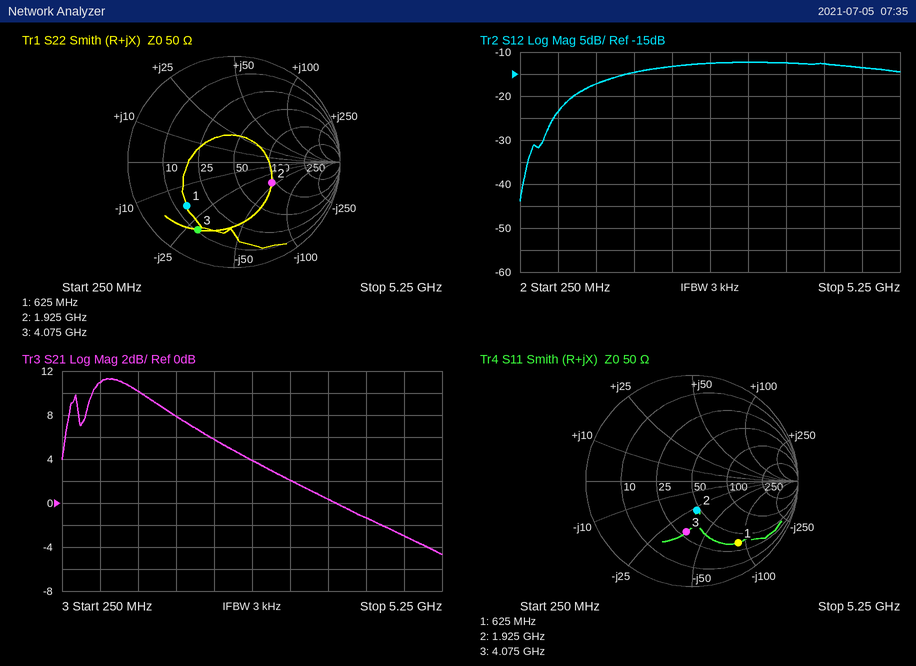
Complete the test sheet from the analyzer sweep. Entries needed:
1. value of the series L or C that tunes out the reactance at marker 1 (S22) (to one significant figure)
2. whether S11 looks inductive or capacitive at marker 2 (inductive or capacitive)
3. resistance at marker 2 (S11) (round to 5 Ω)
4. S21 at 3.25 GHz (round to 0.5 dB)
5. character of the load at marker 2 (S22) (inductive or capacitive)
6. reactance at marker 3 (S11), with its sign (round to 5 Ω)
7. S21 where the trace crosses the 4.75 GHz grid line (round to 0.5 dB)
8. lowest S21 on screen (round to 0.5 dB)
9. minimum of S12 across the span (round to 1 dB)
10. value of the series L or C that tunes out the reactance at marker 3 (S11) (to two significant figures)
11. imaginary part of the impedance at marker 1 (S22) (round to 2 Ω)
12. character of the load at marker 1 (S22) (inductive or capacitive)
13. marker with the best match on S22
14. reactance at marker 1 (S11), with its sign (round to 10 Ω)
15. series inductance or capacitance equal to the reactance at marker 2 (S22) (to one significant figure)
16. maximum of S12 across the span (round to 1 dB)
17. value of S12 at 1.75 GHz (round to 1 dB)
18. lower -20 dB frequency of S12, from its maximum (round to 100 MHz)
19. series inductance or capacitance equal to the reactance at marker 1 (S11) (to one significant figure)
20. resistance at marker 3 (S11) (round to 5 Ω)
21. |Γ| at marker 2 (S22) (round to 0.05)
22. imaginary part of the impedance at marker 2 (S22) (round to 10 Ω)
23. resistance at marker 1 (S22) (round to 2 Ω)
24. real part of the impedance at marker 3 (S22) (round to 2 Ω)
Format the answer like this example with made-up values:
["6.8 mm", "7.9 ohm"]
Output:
["5 nH", "capacitive", "45 Ω", "2.0 dB", "capacitive", "-35 Ω", "-3.0 dB", "-4.5 dB", "-44 dB", "1.4 nH", "-18 Ω", "capacitive", "marker 2", "-90 Ω", "2 pF", "-12 dB", "-15 dB", "400 MHz", "3 pF", "30 Ω", "0.40", "-40 Ω", "14 Ω", "10 Ω"]
